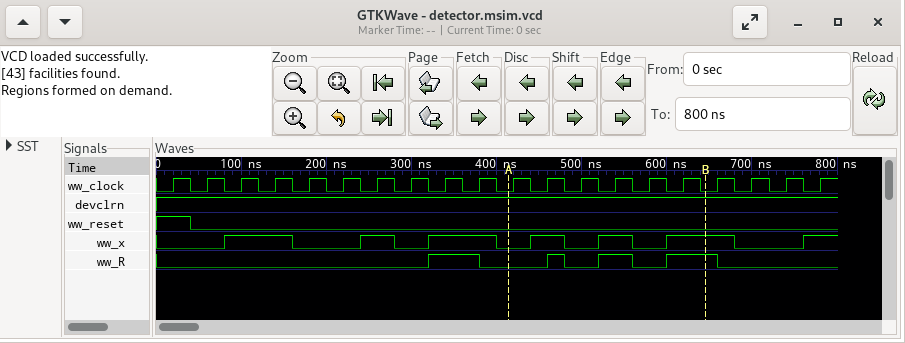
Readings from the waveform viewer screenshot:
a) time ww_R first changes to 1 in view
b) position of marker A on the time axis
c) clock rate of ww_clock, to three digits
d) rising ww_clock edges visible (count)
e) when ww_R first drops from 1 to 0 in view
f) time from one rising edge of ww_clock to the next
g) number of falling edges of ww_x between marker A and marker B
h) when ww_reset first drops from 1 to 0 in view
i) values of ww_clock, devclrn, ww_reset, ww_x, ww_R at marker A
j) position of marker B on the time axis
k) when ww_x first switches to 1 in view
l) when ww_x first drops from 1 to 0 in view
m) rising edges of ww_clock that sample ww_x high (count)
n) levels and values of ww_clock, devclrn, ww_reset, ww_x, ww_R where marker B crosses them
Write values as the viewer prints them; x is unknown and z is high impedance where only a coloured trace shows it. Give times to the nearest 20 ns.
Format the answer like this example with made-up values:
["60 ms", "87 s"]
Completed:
["320 ns", "420 ns", "25.0 MHz", "20", "380 ns", "40 ns", "2", "40 ns", "ww_clock=0, devclrn=1, ww_reset=0, ww_x=0, ww_R=0", "640 ns", "80 ns", "160 ns", "10", "ww_clock=0, devclrn=1, ww_reset=0, ww_x=1, ww_R=1"]
